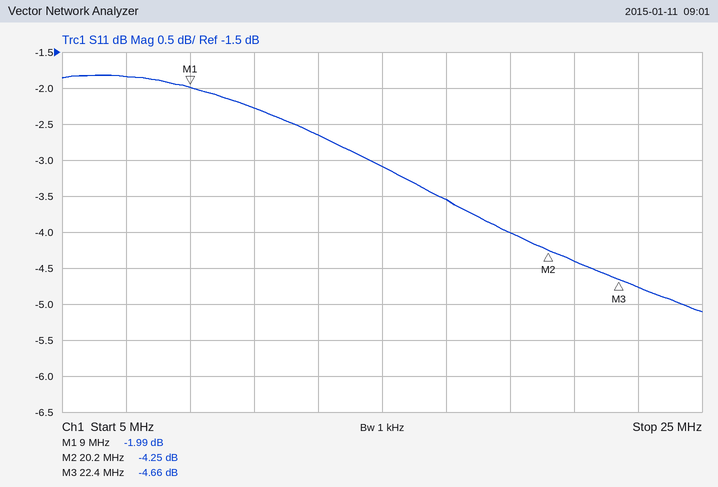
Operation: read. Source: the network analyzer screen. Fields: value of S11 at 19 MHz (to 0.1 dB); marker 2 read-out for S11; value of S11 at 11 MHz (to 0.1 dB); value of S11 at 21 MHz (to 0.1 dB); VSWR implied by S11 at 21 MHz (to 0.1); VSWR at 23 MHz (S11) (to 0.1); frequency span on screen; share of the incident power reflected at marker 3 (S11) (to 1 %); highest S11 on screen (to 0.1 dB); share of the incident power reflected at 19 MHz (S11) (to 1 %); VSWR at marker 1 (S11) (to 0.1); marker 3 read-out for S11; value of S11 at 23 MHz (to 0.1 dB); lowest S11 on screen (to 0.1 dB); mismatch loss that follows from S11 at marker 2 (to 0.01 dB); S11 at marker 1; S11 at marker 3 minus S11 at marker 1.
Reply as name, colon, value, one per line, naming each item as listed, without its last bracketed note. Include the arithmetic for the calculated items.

value of S11 at 19 MHz: -4.0 dB
marker 2 read-out for S11: -4.25 dB
value of S11 at 11 MHz: -2.3 dB
value of S11 at 21 MHz: -4.4 dB
VSWR implied by S11 at 21 MHz: |Γ| = 10^(-4.4/20) = 0.6026; VSWR = (1 + 0.6026)/(1 − 0.6026) ≈ 4.0
VSWR at 23 MHz (S11): |Γ| = 10^(-4.8/20) = 0.5754; VSWR = (1 + 0.5754)/(1 − 0.5754) ≈ 3.7
frequency span on screen: 20 MHz
share of the incident power reflected at marker 3 (S11): 10^(-4.66/10) ≈ 34 %
highest S11 on screen: -1.8 dB
share of the incident power reflected at 19 MHz (S11): 10^(-4/10) ≈ 40 %
VSWR at marker 1 (S11): (1 + 0.7952)/(1 − 0.7952) ≈ 8.8
marker 3 read-out for S11: -4.66 dB
value of S11 at 23 MHz: -4.8 dB
lowest S11 on screen: -5.1 dB
mismatch loss that follows from S11 at marker 2: −10 log10(1 − 10^(-4.25/10)) ≈ 2.05 dB
S11 at marker 1: -1.99 dB
S11 at marker 3 minus S11 at marker 1: -4.66 − (-1.99) = -2.67 dB
